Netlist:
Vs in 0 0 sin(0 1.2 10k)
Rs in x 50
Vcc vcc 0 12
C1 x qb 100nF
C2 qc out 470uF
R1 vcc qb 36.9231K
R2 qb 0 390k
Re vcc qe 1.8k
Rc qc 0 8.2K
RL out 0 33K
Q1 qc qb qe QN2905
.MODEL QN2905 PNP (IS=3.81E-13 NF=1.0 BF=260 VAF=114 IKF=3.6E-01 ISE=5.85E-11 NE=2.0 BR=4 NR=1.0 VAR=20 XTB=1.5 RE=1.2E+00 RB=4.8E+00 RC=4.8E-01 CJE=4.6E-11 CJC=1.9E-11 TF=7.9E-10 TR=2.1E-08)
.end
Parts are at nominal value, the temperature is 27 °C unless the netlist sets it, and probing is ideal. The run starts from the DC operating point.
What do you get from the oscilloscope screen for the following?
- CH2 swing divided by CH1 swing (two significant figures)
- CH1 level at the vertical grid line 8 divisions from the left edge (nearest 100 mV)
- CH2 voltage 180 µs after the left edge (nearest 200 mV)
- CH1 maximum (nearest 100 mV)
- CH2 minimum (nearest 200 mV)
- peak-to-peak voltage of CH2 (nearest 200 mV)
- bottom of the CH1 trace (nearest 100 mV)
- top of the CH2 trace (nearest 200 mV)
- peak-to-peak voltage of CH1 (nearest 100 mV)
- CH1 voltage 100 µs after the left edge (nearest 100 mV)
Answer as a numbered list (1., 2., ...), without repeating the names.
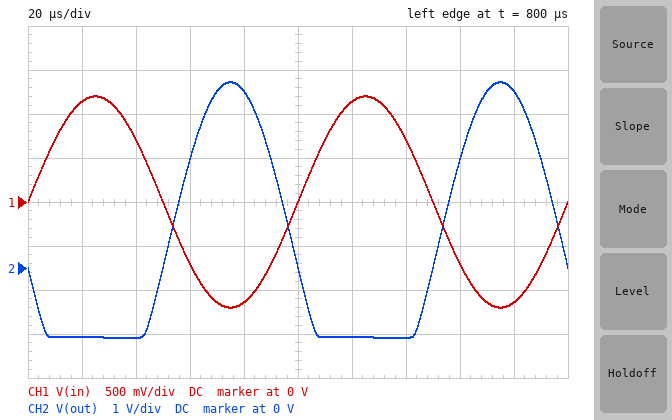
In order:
1. 2.4
2. -700 mV
3. 4.0 V
4. 1.2 V
5. -1.6 V
6. 5.8 V
7. -1.2 V
8. 4.2 V
9. 2.4 V
10. 0 V
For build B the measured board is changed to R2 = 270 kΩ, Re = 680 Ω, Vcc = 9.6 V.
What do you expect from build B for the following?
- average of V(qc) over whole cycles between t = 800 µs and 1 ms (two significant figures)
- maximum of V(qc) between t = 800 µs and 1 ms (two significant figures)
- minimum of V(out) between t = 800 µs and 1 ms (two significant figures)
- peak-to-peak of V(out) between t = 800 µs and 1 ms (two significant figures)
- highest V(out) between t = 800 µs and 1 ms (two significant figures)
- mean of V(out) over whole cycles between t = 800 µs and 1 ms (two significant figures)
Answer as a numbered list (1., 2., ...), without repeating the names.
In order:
1. 3.6 V
2. 8.7 V
3. -4.3 V
4. 7.7 V
5. 3.4 V
6. -1.7 V
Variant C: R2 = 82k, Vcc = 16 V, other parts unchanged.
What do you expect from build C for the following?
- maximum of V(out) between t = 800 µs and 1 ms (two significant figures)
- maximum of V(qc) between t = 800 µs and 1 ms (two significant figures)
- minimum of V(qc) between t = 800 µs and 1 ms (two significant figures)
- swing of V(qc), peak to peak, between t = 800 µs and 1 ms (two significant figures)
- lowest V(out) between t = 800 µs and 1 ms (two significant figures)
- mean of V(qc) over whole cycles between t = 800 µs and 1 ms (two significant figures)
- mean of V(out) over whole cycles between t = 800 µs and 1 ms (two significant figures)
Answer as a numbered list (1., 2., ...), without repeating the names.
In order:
1. 30 mV
2. 13 V
3. 6.7 V
4. 6.3 V
5. -6.3 V
6. 10 V
7. -2.6 V
